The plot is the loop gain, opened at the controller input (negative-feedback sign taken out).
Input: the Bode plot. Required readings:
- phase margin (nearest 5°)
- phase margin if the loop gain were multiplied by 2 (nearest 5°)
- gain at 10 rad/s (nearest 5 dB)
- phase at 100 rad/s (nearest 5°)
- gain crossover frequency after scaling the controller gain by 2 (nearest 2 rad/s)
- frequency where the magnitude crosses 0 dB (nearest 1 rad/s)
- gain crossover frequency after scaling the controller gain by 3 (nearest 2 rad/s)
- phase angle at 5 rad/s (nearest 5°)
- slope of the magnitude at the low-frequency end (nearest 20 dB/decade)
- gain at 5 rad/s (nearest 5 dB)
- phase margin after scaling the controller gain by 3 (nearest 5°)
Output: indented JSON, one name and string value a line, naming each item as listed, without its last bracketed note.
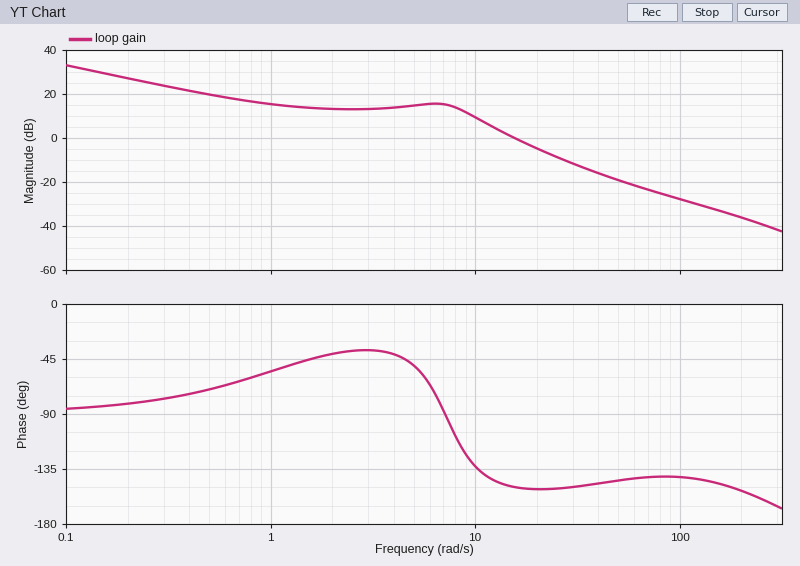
{
  "phase margin": "30°",
  "phase margin if the loop gain were multiplied by 2": "30°",
  "gain at 10 rad/s": "10 dB",
  "phase at 100 rad/s": "-140°",
  "gain crossover frequency after scaling the controller gain by 2": "22 rad/s",
  "frequency where the magnitude crosses 0 dB": "16 rad/s",
  "gain crossover frequency after scaling the controller gain by 3": "26 rad/s",
  "phase angle at 5 rad/s": "-50°",
  "slope of the magnitude at the low-frequency end": "-20 dB/decade",
  "gain at 5 rad/s": "15 dB",
  "phase margin after scaling the controller gain by 3": "30°"
}
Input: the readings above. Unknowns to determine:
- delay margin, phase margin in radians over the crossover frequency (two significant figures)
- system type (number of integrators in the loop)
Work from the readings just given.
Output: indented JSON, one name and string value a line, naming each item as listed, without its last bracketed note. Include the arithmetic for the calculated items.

{
  "delay margin, phase margin in radians over the crossover frequency": "30 × π / 180 / 16 = 0.033 s",
  "system type": "1"
}
